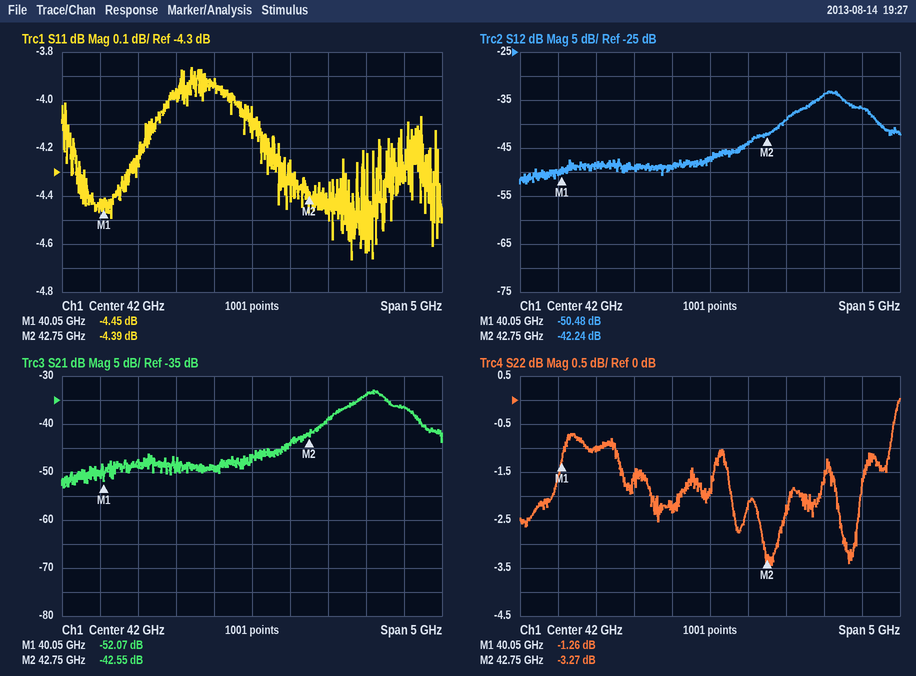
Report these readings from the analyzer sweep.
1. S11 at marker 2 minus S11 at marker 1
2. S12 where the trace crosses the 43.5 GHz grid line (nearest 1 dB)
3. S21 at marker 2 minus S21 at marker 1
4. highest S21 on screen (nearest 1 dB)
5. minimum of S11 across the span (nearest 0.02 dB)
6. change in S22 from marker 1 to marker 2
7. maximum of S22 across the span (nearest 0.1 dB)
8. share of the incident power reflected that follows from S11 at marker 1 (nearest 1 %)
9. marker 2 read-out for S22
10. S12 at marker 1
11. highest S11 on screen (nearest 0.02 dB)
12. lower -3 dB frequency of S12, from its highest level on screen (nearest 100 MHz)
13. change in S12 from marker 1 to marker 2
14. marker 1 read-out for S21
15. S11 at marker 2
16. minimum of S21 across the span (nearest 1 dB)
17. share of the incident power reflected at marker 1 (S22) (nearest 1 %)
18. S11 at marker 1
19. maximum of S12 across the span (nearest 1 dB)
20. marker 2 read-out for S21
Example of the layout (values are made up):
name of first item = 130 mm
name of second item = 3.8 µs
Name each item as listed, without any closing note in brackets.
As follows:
S11 at marker 2 minus S11 at marker 1 = 0.06 dB
S12 where the trace crosses the 43.5 GHz grid line = -34 dB
S21 at marker 2 minus S21 at marker 1 = 9.52 dB
highest S21 on screen = -33 dB
minimum of S11 across the span = -4.66 dB
change in S22 from marker 1 to marker 2 = -2.01 dB
maximum of S22 across the span = 0.0 dB
share of the incident power reflected that follows from S11 at marker 1 = 36 %
marker 2 read-out for S22 = -3.27 dB
S12 at marker 1 = -50.48 dB
highest S11 on screen = -3.86 dB
lower -3 dB frequency of S12, from its highest level on screen = 43.3 GHz
change in S12 from marker 1 to marker 2 = 8.24 dB
marker 1 read-out for S21 = -52.07 dB
S11 at marker 2 = -4.39 dB
minimum of S21 across the span = -53 dB
share of the incident power reflected at marker 1 (S22) = 75 %
S11 at marker 1 = -4.45 dB
maximum of S12 across the span = -33 dB
marker 2 read-out for S21 = -42.55 dB
